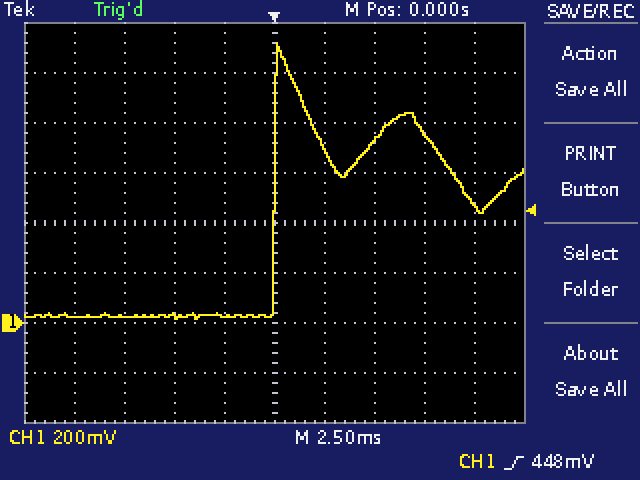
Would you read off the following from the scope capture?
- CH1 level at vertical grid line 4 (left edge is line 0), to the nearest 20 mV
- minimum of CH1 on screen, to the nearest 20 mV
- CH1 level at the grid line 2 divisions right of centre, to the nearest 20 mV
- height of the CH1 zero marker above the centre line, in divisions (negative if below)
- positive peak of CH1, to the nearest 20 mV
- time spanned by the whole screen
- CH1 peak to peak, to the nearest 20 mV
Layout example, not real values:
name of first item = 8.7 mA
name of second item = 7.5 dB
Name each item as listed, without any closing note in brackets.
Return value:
CH1 level at vertical grid line 4 (left edge is line 0), to the nearest 20 mV = 20 mV
minimum of CH1 on screen, to the nearest 20 mV = 20 mV
CH1 level at the grid line 2 divisions right of centre, to the nearest 20 mV = 720 mV
height of the CH1 zero marker above the centre line, in divisions = -2.0 div
positive peak of CH1, to the nearest 20 mV = 1.12 V
time spanned by the whole screen = 25 ms
CH1 peak to peak, to the nearest 20 mV = 1.10 V
